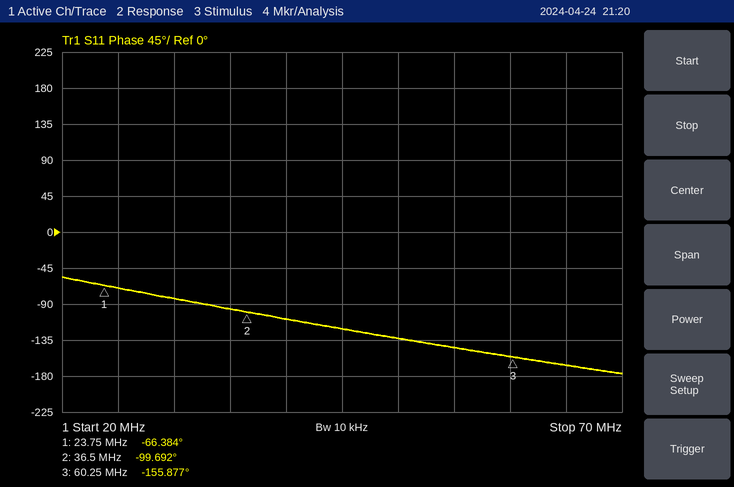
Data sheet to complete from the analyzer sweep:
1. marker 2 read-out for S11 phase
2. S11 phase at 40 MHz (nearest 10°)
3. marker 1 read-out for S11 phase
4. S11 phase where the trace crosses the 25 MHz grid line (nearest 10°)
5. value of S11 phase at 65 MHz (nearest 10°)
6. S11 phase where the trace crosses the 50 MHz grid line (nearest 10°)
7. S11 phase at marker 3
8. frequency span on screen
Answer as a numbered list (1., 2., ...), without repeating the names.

1. -99.692°
2. -110°
3. -66.384°
4. -70°
5. -170°
6. -130°
7. -155.877°
8. 50 MHz
